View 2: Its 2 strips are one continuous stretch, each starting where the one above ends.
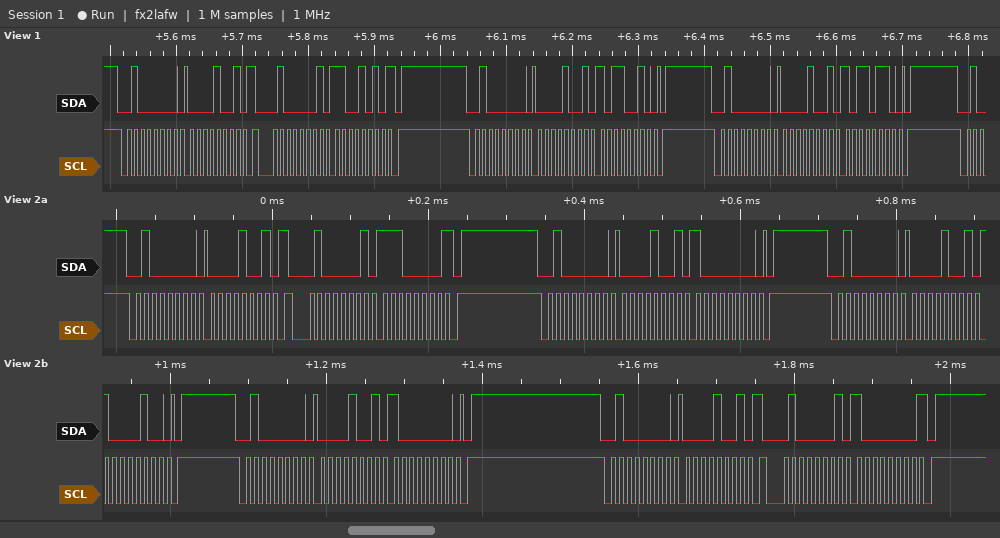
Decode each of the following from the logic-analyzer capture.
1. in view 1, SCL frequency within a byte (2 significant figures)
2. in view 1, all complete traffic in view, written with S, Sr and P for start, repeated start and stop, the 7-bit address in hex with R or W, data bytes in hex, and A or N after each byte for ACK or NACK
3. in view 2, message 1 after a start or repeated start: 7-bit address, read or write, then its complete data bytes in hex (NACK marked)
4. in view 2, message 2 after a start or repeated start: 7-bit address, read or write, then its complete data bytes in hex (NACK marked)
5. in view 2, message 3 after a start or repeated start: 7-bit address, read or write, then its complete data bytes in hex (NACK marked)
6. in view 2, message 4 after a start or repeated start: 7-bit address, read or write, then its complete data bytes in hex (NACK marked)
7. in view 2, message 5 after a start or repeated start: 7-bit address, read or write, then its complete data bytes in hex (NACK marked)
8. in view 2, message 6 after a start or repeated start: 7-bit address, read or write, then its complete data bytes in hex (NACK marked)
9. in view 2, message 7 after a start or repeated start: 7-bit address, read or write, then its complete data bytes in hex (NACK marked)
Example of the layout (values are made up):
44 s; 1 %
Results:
100 kHz; S 20W A 09 A Sr 20R A CA N P S 20W A 09 A B2 A P S 20W A 09 A B6 A P; 0x20 write: 09; 0x20 read: E0 NACK; 0x20 write: 09 80; 0x20 write: 09 84; 0x20 write: 09 80; 0x20 write: 09; 0x20 read: 80 NACK
